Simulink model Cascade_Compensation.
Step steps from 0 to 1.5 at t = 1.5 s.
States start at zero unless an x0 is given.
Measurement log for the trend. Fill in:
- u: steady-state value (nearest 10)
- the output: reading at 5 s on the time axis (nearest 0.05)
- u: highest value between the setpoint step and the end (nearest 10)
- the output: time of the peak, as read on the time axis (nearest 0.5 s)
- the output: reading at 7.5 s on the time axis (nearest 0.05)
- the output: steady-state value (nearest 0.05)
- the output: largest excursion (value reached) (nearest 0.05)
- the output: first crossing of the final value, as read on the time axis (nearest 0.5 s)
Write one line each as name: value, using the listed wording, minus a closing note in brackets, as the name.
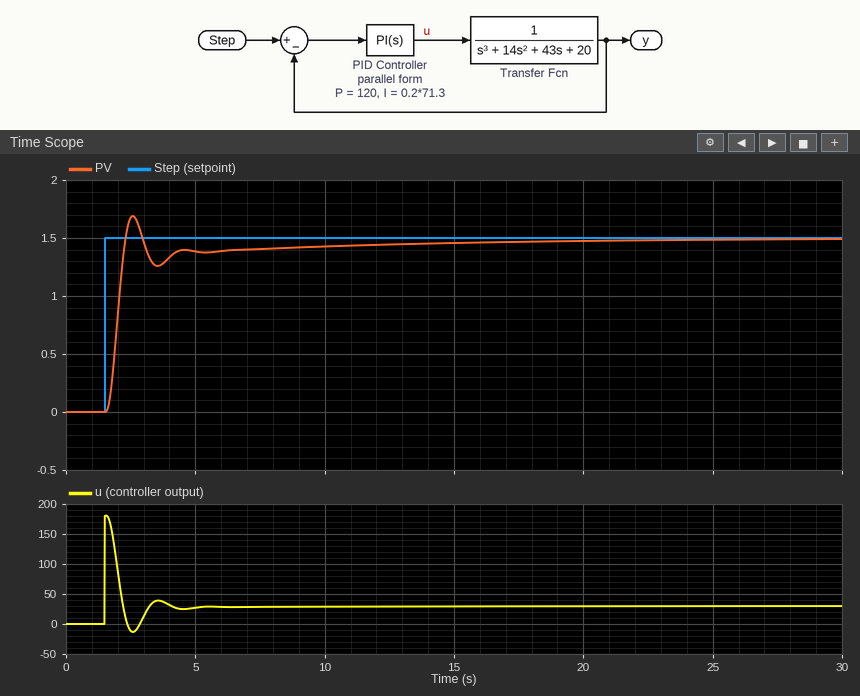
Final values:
u: steady-state value: 30
the output: reading at 5 s on the time axis: 1.40
u: highest value between the setpoint step and the end: 180
the output: time of the peak, as read on the time axis: 2.5 s
the output: reading at 7.5 s on the time axis: 1.40
the output: steady-state value: 1.50
the output: largest excursion (value reached): 1.70
the output: first crossing of the final value, as read on the time axis: 2.5 s
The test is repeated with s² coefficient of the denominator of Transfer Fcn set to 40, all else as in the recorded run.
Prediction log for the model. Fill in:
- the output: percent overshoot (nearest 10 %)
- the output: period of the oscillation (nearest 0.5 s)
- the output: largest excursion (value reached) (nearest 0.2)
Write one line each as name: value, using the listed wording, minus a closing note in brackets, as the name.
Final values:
the output: percent overshoot: 30 %
the output: period of the oscillation: 3.5 s
the output: largest excursion (value reached): 2.0
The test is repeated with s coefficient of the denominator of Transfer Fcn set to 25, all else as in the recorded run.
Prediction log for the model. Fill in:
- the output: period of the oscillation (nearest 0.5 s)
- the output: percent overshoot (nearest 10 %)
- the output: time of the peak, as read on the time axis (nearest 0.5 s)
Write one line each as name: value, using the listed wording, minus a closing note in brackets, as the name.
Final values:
the output: period of the oscillation: 2.0 s
the output: percent overshoot: 40 %
the output: time of the peak, as read on the time axis: 2.5 s
